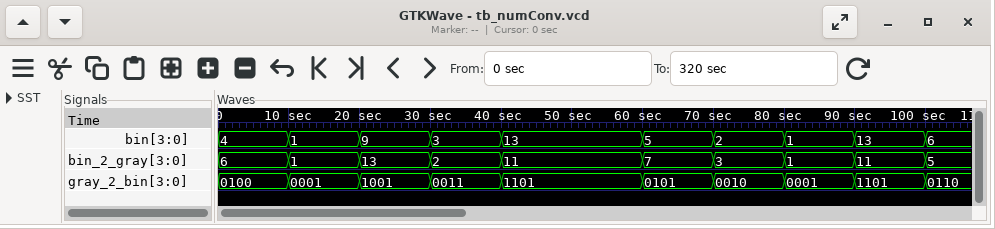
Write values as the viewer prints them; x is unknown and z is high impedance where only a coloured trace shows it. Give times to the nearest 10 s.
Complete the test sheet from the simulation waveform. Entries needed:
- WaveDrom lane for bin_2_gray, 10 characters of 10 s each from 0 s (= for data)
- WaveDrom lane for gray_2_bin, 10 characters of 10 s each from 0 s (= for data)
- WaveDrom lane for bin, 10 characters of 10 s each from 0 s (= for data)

{name: 'bin_2_gray', wave: '=====.====', data: '6 1 13 2 11 7 3 1 11'}
{name: 'gray_2_bin', wave: '=====.====', data: '0100 0001 1001 0011 1101 0101 0010 0001 1101'}
{name: 'bin', wave: '=====.====', data: '4 1 9 3 13 5 2 1 13'}
